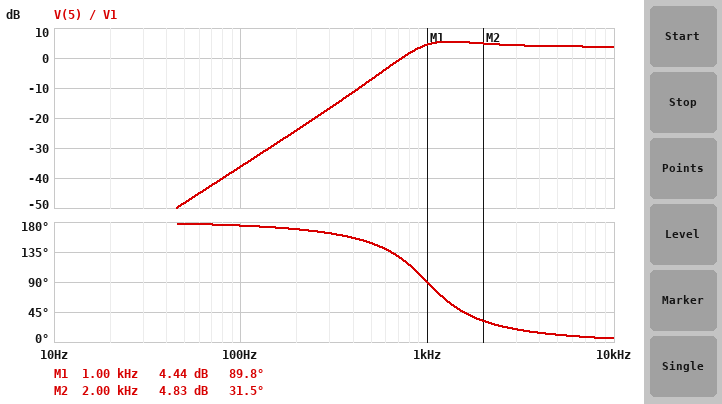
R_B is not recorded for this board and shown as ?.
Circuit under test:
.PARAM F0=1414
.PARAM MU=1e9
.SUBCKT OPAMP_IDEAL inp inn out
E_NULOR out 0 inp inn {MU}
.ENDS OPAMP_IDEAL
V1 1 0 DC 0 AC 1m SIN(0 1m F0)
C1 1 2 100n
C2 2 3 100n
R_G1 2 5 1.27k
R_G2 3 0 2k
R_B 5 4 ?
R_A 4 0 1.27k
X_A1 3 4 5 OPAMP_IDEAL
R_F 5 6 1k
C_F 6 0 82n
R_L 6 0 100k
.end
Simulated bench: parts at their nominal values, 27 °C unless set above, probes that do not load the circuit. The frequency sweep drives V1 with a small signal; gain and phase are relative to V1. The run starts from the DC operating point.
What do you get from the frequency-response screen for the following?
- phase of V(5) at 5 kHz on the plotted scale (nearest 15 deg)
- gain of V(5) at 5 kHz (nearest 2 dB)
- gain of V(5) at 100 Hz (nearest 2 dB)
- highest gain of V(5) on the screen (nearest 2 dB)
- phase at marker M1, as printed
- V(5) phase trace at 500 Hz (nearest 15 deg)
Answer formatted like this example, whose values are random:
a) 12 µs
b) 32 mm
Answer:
a) 15 deg
b) 4 dB
c) -36 dB
d) 6 dB
e) 89.8 deg
f) 150 deg
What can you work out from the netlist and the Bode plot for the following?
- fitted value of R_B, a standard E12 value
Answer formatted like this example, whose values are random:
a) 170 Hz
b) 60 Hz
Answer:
a) 680 Ω
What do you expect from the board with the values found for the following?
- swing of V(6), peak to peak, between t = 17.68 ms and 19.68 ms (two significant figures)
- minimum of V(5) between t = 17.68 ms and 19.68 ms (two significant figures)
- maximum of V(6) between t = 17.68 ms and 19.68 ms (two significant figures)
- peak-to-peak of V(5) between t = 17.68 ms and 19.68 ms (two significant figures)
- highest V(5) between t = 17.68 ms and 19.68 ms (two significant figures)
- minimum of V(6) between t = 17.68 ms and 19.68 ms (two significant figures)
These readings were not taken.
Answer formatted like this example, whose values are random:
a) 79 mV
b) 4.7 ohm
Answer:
a) 3.0 mV
b) -1.9 mV
c) 1.5 mV
d) 3.7 mV
e) 1.9 mV
f) -1.5 mV
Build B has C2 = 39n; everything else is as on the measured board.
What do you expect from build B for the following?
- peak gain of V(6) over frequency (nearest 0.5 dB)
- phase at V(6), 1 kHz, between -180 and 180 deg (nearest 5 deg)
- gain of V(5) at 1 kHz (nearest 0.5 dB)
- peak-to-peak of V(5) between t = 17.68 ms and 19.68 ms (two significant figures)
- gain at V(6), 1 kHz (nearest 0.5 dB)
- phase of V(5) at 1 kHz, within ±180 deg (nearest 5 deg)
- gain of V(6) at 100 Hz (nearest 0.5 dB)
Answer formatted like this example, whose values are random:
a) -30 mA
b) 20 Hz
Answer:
a) -0.5 dB
b) 100 deg
c) -5.0 dB
d) 2.0 mV
e) -6.0 dB
f) 125 deg
g) -44.5 dB
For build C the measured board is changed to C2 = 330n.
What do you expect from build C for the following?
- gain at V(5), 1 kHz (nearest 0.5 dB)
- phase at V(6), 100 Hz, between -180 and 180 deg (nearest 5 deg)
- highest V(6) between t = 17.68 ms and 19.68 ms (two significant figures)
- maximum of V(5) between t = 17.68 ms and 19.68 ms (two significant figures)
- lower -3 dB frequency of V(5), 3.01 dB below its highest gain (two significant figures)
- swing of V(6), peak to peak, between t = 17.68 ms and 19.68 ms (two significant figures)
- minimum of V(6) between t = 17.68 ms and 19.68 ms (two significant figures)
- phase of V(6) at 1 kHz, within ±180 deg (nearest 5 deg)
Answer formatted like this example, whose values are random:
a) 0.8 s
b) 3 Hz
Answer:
a) 6.0 dB
b) 170 deg
c) 1.4 mV
d) 1.7 mV
e) 460 Hz
f) 2.8 mV
g) -1.4 mV
h) 0 deg
